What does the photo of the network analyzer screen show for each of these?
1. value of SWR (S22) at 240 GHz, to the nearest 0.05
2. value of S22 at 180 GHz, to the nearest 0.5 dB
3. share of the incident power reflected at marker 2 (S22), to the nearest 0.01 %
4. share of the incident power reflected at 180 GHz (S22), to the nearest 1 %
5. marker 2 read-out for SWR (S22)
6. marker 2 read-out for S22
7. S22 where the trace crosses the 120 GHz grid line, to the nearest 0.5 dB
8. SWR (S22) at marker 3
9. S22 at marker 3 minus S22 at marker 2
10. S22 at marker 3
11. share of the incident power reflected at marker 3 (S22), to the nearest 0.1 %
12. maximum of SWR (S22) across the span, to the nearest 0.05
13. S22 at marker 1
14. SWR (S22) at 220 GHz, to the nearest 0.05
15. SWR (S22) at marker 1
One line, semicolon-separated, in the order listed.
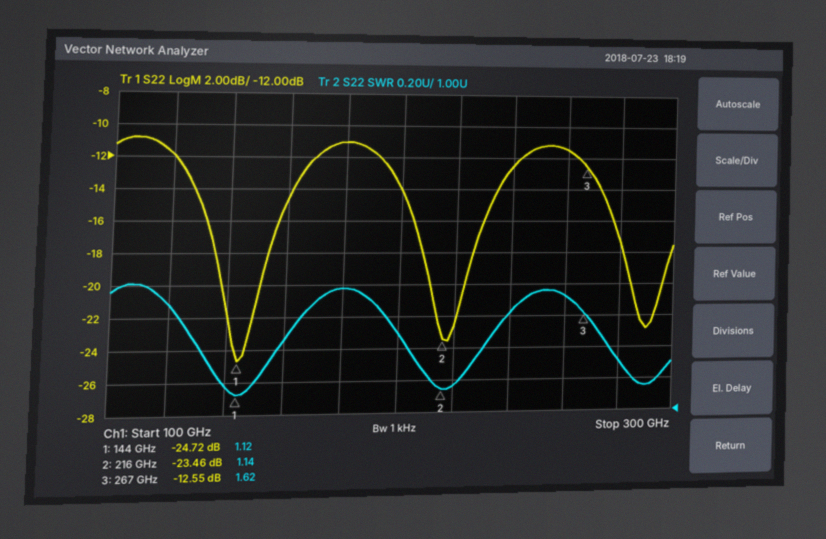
1.60; -11.0 dB; 0.45 %; 8 %; 1.14; -23.46 dB; -12.0 dB; 1.62; 10.91 dB; -12.55 dB; 5.6 %; 1.80; -24.72 dB; 1.15; 1.12
